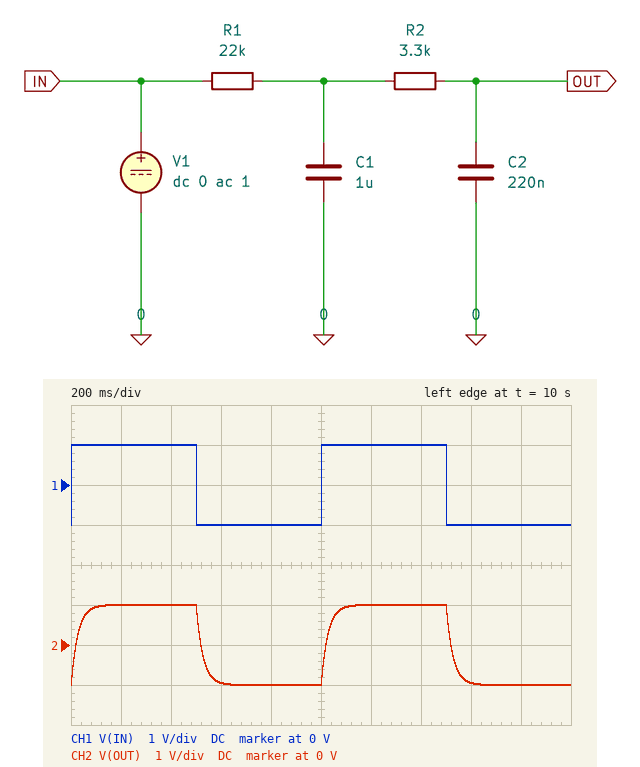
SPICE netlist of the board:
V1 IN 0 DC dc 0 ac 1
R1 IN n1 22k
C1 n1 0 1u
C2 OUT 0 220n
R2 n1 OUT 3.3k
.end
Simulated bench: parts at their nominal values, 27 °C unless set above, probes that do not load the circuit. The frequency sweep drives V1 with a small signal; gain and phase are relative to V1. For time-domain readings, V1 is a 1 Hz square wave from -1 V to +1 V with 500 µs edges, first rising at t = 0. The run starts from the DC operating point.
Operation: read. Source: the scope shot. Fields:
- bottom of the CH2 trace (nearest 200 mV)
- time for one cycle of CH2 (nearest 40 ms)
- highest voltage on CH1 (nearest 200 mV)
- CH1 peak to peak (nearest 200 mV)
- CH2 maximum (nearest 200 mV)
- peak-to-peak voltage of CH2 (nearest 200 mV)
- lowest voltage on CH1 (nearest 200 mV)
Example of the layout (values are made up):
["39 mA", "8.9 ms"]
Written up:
["-1.0 V", "1.00 s", "1.0 V", "2.0 V", "1.0 V", "2.0 V", "-1.0 V"]
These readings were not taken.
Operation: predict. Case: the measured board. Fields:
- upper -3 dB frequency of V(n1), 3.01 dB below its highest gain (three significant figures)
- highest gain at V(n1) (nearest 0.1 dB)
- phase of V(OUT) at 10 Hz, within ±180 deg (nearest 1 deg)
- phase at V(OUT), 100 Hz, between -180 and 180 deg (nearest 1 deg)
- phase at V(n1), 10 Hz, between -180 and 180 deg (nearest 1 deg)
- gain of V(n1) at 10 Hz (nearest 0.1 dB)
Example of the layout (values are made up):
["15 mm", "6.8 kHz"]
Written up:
["5.90 Hz", "0 dB", "-62 deg", "-107 deg", "-59 deg", "-5.9 dB"]
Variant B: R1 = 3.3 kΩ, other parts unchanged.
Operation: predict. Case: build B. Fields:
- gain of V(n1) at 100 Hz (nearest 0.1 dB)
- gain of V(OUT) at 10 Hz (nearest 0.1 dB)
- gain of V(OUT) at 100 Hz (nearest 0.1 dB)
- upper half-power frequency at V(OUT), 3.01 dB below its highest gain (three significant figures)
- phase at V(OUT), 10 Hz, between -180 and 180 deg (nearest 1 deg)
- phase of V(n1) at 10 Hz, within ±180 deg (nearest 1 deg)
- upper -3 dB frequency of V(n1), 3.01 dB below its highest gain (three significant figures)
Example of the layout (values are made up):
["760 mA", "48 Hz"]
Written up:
["-8.7 dB", "-0.3 dB", "-9.5 dB", "37.4 Hz", "-17 deg", "-14 deg", "38.5 Hz"]
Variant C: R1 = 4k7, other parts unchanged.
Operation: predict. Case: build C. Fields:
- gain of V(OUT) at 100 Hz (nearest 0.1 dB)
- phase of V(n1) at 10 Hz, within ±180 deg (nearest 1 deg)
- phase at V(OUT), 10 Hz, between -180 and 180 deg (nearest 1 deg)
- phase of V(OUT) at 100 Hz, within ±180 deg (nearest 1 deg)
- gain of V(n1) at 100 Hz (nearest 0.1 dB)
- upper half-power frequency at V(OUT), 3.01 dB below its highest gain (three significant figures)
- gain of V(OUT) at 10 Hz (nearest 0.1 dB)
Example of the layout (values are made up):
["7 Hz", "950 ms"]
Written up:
["-12.2 dB", "-20 deg", "-22 deg", "-95 deg", "-11.4 dB", "26.8 Hz", "-0.6 dB"]
